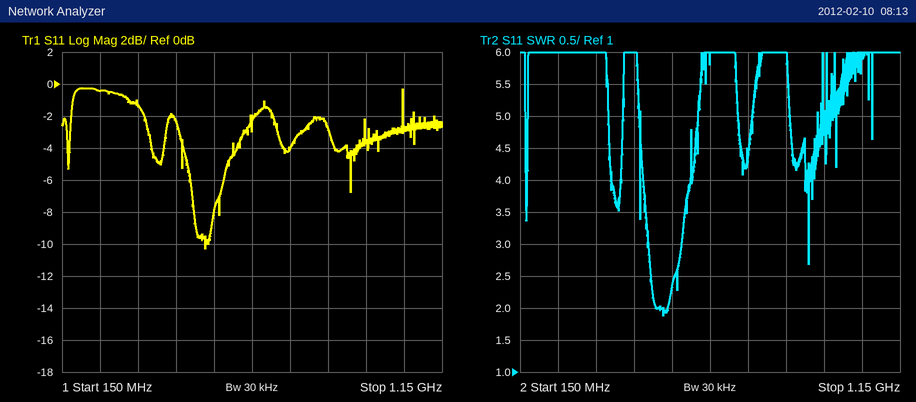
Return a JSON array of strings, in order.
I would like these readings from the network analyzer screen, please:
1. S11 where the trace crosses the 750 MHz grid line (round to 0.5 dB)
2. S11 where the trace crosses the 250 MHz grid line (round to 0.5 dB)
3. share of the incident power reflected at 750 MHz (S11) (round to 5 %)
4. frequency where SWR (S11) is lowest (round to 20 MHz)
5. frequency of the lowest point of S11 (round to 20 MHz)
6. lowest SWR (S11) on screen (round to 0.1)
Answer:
["-4.0 dB", "-0.5 dB", "40 %", "520 MHz", "520 MHz", "1.9"]
